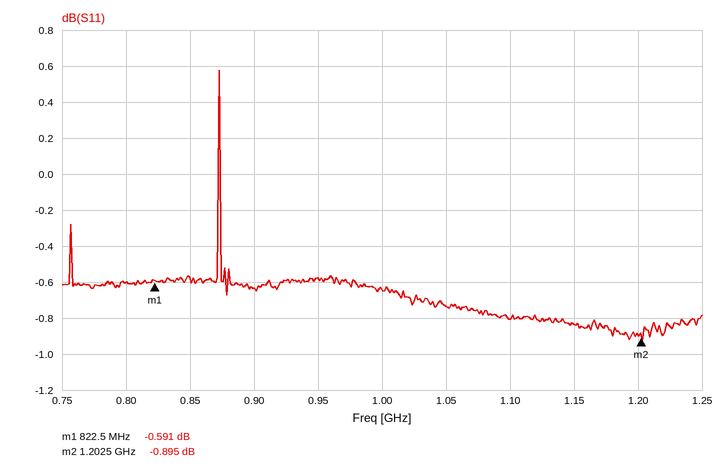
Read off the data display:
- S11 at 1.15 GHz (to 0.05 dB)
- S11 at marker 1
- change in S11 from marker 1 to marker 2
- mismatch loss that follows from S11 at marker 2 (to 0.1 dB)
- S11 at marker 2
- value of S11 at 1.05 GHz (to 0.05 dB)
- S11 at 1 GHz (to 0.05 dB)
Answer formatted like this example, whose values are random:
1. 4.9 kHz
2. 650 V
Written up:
1. -0.85 dB
2. -0.591 dB
3. -0.304 dB
4. 7.3 dB
5. -0.895 dB
6. -0.75 dB
7. -0.65 dB
